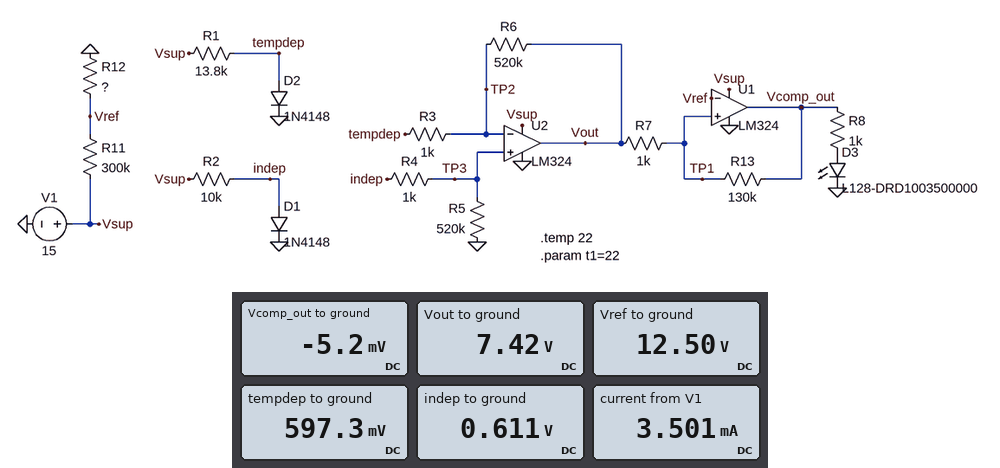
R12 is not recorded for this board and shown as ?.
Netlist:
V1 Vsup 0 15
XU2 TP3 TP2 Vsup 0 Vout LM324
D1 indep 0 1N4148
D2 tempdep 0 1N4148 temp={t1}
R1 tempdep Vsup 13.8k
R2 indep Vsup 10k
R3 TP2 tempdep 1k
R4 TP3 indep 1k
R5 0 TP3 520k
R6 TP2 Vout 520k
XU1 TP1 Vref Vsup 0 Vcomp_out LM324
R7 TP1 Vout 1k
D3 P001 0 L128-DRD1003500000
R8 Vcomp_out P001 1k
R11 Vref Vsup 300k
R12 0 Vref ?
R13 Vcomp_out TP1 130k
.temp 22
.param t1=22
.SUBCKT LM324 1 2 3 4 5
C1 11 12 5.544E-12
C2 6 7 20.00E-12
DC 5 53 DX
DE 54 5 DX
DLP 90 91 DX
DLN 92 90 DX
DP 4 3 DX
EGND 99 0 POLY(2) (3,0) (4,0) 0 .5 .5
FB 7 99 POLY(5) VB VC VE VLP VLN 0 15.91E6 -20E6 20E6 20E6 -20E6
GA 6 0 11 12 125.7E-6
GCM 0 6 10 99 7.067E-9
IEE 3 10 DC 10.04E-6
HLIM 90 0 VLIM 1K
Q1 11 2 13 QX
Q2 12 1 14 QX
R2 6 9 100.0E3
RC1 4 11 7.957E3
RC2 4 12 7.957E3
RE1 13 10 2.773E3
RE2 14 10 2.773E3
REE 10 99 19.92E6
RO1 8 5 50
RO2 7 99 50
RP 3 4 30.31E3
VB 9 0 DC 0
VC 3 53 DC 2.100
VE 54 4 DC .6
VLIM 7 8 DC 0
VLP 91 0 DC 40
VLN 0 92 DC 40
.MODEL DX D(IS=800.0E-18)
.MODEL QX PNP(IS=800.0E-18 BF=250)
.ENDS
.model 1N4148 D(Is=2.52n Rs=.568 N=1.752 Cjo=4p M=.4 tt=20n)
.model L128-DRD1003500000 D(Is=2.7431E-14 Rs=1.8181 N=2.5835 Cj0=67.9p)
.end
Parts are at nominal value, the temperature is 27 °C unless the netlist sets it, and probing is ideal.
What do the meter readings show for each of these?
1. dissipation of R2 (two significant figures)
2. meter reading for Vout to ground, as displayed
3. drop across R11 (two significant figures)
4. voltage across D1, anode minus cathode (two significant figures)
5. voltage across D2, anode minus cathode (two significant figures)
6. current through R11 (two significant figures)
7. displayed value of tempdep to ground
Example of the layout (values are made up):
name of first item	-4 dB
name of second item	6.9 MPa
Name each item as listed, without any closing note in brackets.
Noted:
dissipation of R2	21 mW
meter reading for Vout to ground, as displayed	7.42 V
drop across R11	2.5 V
voltage across D1, anode minus cathode	610 mV
voltage across D2, anode minus cathode	600 mV
current through R11	8.3 µA
displayed value of tempdep to ground	597.3 mV
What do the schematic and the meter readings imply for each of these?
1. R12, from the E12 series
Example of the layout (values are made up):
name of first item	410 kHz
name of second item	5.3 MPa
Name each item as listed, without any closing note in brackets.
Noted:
R12, from the E12 series	1.5 MΩ
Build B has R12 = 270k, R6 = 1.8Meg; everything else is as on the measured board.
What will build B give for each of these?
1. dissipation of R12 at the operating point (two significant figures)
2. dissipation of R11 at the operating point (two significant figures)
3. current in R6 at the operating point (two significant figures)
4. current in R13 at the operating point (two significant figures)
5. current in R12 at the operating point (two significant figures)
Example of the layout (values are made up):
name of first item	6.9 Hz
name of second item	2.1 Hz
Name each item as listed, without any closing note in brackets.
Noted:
dissipation of R12 at the operating point	190 µW
dissipation of R11 at the operating point	210 µW
current in R6 at the operating point	7.1 µA
current in R13 at the operating point	490 nA
current in R12 at the operating point	26 µA
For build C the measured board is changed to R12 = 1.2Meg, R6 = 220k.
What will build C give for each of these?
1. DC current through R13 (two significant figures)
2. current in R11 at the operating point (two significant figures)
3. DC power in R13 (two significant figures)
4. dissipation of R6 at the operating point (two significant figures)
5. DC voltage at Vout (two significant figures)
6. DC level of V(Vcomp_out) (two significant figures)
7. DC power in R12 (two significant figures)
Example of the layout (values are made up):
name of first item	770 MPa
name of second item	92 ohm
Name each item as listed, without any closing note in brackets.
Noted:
DC current through R13	27 µA
current in R11 at the operating point	10 µA
DC power in R13	93 µW
dissipation of R6 at the operating point	38 µW
DC voltage at Vout	3.5 V
DC level of V(Vcomp_out)	-5.6 mV
DC power in R12	120 µW
